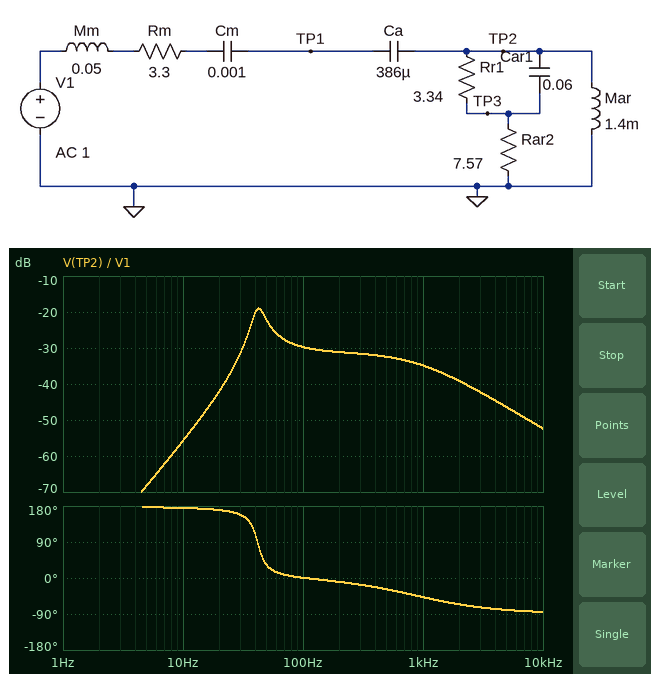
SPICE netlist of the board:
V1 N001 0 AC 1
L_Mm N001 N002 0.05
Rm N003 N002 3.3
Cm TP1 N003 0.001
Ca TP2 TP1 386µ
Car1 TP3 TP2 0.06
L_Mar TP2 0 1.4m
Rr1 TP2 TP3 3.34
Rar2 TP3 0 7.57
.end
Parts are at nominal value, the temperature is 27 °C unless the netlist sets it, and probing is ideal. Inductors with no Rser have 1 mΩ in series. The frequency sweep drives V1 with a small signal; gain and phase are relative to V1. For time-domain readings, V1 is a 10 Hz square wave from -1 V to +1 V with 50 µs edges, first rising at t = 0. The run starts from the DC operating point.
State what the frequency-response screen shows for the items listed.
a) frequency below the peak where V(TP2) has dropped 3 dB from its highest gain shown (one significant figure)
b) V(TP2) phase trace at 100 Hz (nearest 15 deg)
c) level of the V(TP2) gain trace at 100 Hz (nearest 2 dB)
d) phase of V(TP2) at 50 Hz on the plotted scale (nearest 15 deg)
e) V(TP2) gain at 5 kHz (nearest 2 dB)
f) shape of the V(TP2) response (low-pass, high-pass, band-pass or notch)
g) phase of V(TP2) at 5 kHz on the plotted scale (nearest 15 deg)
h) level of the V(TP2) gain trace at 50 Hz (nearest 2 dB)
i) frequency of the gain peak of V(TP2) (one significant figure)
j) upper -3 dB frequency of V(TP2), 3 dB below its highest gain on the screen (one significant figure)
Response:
40 Hz
0 deg
-30 dB
30 deg
-46 dB
band-pass
-75 deg
-22 dB
40 Hz
50 Hz
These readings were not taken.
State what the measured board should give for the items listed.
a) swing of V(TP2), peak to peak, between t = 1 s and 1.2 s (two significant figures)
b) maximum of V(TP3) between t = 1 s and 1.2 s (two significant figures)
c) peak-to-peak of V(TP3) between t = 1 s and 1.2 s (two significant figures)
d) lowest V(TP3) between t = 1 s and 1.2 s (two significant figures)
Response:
89 mV
44 mV
89 mV
-44 mV
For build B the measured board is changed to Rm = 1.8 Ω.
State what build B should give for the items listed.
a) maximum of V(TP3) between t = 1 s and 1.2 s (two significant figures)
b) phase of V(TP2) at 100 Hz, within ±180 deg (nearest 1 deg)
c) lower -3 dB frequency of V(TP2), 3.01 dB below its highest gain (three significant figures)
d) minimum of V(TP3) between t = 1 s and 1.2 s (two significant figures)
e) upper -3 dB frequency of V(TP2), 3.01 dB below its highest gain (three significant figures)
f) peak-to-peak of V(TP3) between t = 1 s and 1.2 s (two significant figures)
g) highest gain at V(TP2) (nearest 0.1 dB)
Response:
39 mV
-3 deg
39.7 Hz
-39 mV
45.4 Hz
79 mV
-13.8 dB
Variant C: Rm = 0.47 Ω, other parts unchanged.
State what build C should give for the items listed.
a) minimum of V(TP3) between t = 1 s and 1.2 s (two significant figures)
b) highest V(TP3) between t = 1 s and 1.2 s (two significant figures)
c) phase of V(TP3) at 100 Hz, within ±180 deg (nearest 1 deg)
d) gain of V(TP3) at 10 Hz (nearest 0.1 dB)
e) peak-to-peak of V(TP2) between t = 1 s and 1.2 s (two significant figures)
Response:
-32 mV
32 mV
-5 deg
-55.8 dB
64 mV
